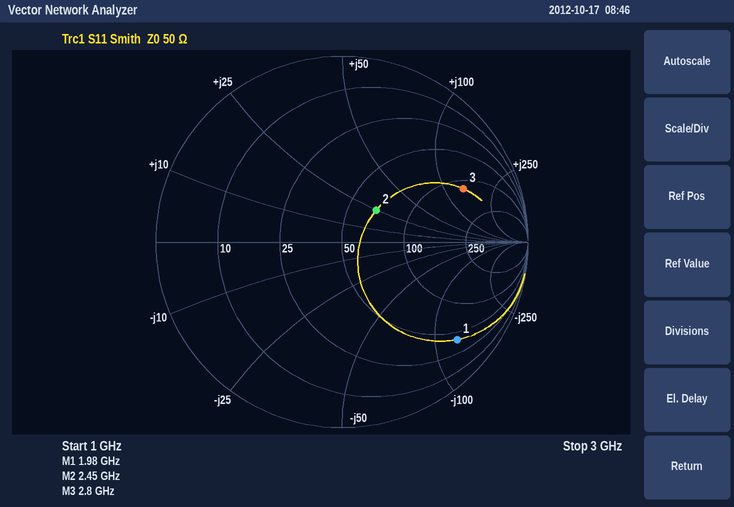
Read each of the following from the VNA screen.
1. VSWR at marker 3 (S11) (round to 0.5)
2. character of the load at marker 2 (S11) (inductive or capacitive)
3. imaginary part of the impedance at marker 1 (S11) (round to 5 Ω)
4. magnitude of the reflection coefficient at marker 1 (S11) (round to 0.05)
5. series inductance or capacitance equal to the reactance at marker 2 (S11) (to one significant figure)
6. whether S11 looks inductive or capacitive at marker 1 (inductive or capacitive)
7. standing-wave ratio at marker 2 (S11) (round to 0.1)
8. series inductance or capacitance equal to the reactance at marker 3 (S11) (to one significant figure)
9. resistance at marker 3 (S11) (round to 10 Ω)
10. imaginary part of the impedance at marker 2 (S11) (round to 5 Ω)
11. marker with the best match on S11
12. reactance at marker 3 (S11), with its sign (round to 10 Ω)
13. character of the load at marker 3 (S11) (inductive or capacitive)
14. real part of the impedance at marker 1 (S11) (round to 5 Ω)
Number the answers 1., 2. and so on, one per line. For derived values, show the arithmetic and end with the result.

1. 6.0
2. inductive
3. -125 Ω
4. 0.80
5. L = 25 Ω/(2π × 2.45 GHz) ≈ 2 nH
6. capacitive
7. 1.7
8. L = 140 Ω/(2π × 2.8 GHz) ≈ 8 nH
9. 120 Ω
10. +25 Ω
11. marker 2
12. +140 Ω
13. inductive
14. 40 Ω
